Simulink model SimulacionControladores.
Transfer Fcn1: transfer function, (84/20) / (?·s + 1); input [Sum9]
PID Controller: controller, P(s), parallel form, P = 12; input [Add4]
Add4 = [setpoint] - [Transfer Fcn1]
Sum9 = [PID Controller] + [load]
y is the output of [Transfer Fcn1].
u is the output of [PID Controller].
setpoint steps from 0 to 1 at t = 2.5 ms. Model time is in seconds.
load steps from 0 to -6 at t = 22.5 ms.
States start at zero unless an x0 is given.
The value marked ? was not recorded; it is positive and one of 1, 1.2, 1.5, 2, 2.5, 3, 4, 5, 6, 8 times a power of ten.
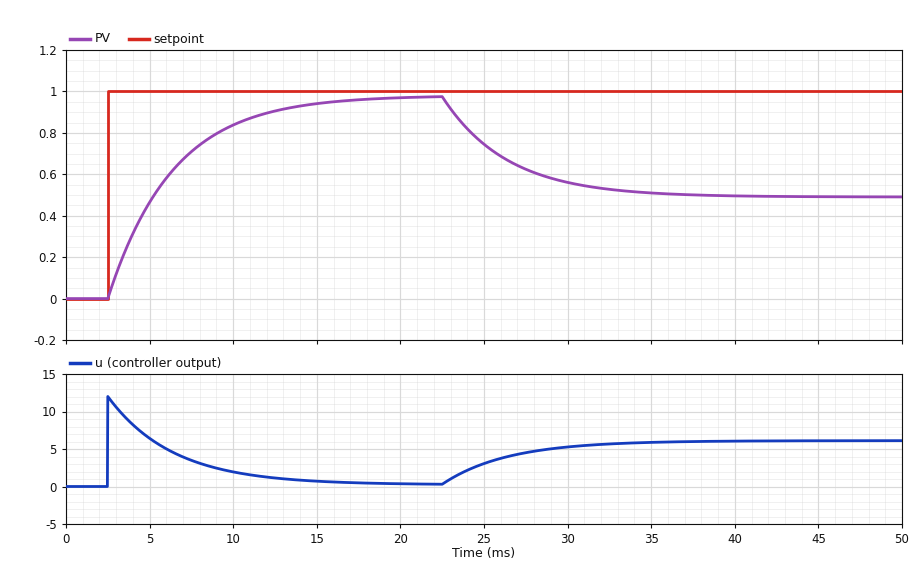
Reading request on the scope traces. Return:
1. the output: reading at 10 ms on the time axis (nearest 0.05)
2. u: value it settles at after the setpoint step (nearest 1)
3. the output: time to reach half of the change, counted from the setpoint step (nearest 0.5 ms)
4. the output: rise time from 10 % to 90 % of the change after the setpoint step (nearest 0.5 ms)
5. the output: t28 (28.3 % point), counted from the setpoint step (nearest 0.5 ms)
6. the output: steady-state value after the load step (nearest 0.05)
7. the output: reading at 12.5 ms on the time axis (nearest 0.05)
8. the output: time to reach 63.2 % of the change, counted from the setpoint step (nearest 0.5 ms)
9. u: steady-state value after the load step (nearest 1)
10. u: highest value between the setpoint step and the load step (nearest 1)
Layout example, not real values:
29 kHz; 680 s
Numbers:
0.85; 0; 2.5 ms; 8.5 ms; 1.5 ms; 0.50; 0.90; 4.0 ms; 6; 12
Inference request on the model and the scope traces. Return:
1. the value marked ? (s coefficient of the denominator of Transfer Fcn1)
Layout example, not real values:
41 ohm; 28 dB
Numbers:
0.2
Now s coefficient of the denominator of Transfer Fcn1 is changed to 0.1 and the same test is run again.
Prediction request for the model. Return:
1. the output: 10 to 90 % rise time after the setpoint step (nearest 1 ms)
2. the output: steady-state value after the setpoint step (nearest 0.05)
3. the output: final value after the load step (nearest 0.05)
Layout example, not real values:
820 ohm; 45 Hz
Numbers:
4 ms; 1.00; 0.50
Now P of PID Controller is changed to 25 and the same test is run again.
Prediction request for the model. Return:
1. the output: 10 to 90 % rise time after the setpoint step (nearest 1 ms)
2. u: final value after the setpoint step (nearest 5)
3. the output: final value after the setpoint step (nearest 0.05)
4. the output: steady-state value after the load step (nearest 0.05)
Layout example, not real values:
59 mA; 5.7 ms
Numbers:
4 ms; 0; 1.00; 0.75
